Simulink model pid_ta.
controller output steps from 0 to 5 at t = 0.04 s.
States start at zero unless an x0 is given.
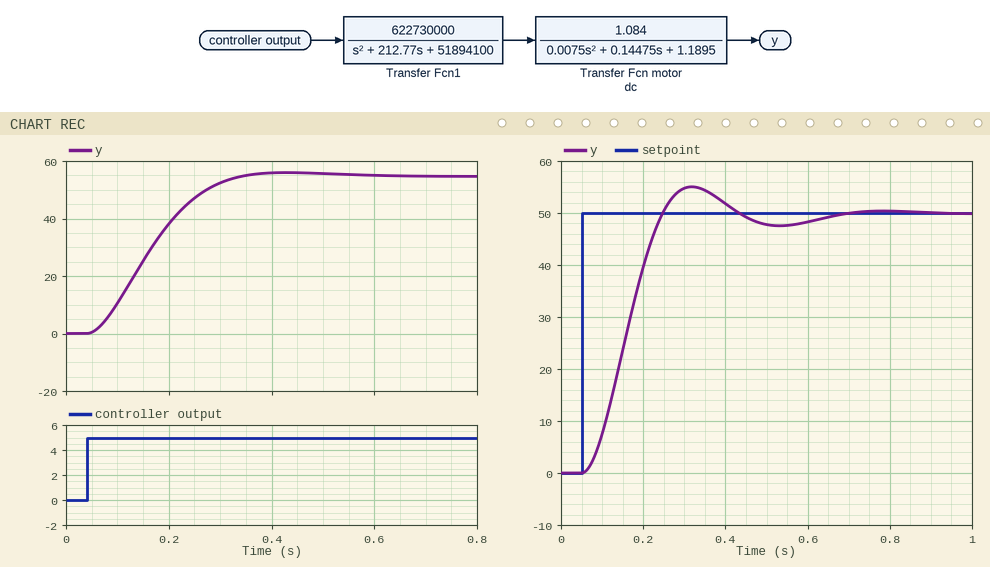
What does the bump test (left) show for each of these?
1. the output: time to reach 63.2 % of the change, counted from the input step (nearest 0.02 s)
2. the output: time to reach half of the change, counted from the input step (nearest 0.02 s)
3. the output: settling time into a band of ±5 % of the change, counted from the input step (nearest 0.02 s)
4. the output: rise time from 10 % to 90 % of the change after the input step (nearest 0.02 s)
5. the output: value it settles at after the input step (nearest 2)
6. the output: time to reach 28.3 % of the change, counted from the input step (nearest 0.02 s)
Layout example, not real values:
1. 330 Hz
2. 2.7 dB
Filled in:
1. 0.14 s
2. 0.12 s
3. 0.26 s
4. 0.18 s
5. 54
6. 0.08 s
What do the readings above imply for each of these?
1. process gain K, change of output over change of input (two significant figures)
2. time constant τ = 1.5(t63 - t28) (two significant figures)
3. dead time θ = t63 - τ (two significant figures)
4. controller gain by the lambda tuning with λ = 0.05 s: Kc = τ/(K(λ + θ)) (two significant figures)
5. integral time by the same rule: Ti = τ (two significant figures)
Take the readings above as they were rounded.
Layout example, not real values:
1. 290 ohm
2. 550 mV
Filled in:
1. 11
2. 0.090 s
3. 0.050 s
4. 0.082
5. 0.090 s
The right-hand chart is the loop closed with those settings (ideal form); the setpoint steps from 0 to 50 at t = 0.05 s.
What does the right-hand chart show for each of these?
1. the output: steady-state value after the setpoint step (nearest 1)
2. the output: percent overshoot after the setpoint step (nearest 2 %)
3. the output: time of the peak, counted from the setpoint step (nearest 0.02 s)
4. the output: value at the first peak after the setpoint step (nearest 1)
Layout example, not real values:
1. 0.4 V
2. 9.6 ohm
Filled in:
1. 50
2. 10 %
3. 0.26 s
4. 55
